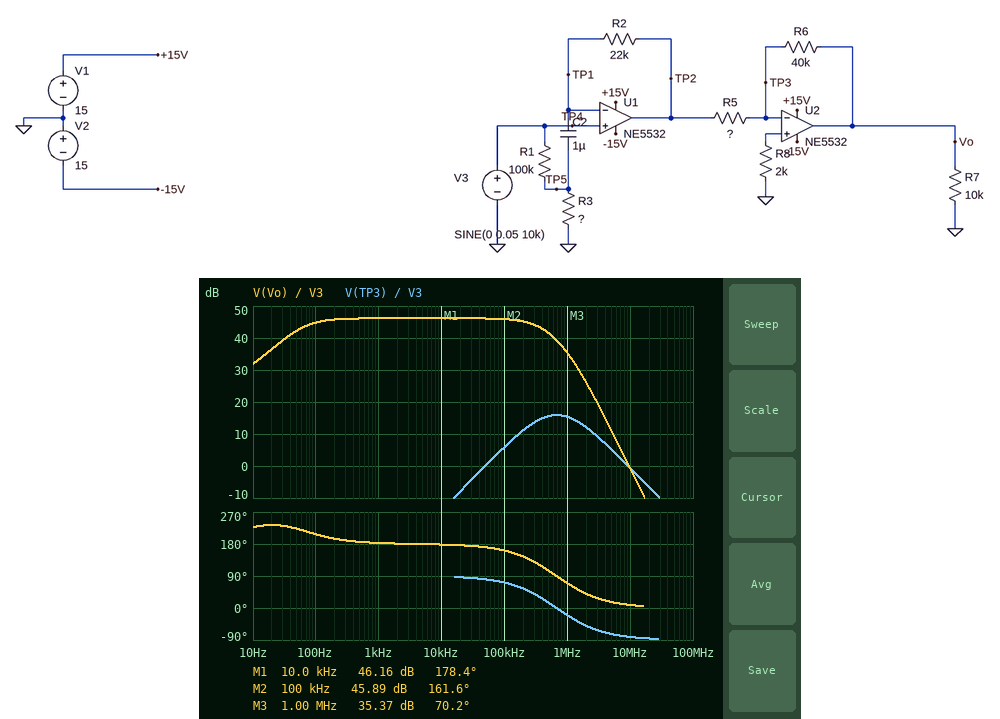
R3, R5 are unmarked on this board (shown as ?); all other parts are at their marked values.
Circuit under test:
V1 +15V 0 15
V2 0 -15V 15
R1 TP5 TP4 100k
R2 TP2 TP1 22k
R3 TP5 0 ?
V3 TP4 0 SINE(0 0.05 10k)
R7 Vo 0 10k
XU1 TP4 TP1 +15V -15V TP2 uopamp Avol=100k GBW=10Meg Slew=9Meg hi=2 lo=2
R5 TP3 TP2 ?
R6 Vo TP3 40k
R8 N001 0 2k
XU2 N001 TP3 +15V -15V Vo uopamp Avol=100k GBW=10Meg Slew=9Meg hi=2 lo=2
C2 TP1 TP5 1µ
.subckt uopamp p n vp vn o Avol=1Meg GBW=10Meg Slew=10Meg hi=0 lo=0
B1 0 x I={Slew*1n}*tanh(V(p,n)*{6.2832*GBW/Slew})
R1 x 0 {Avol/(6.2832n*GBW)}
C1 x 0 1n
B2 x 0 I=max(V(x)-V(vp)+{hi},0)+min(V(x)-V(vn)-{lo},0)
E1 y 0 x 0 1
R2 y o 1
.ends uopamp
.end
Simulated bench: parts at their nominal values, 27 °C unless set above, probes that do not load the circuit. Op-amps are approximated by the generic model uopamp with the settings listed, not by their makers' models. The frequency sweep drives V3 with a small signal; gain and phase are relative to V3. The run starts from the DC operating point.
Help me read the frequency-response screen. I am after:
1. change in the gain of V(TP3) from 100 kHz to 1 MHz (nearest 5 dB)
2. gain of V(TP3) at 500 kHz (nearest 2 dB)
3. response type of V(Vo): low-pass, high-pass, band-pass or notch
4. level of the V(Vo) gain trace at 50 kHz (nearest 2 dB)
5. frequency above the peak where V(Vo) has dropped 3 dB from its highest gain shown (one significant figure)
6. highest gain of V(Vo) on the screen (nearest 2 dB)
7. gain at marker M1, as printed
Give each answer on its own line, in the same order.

10 dB
16 dB
band-pass
46 dB
400 kHz
46 dB
46.16 dB
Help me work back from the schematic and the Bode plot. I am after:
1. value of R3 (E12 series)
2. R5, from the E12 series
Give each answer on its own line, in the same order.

2.7 kΩ
1.8 kΩ
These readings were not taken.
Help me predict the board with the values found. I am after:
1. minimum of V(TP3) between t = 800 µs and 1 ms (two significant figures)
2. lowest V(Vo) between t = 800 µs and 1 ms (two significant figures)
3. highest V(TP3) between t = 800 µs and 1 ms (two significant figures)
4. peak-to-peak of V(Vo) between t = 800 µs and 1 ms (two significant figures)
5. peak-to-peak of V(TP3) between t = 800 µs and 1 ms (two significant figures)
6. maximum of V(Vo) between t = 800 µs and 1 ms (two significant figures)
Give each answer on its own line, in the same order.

-10 mV
-10 V
10 mV
20 V
20 mV
10 V
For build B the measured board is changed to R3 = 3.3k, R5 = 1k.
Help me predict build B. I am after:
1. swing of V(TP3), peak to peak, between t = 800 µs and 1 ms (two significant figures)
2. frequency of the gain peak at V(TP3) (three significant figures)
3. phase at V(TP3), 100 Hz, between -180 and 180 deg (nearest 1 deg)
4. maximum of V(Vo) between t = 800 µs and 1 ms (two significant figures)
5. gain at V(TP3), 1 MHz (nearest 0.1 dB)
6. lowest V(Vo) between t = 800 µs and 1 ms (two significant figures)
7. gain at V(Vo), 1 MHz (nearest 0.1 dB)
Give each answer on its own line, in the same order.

110 mV
556 kHz
68 deg
13 V
15.1 dB
-13 V
35.1 dB
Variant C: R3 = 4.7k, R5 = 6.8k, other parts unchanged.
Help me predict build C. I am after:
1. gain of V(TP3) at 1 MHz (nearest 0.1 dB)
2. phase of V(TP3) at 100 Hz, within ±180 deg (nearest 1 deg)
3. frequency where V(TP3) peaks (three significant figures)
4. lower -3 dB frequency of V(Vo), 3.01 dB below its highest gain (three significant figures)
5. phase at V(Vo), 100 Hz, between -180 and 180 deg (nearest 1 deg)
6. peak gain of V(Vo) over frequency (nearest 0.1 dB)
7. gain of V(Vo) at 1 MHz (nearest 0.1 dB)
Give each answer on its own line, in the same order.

7.5 dB
61 deg
1.57 MHz
34.3 Hz
-164 deg
30.5 dB
27.5 dB
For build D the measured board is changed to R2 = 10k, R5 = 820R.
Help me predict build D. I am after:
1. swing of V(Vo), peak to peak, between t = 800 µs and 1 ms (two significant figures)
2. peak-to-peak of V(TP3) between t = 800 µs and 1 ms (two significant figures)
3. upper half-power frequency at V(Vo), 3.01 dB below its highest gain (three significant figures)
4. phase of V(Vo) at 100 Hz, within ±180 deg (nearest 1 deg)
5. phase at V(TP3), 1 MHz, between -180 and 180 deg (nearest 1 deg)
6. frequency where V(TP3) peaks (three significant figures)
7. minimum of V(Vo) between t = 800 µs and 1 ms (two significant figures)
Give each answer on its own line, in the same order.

23 V
23 mV
199 kHz
-156 deg
-14 deg
647 kHz
-11 V
